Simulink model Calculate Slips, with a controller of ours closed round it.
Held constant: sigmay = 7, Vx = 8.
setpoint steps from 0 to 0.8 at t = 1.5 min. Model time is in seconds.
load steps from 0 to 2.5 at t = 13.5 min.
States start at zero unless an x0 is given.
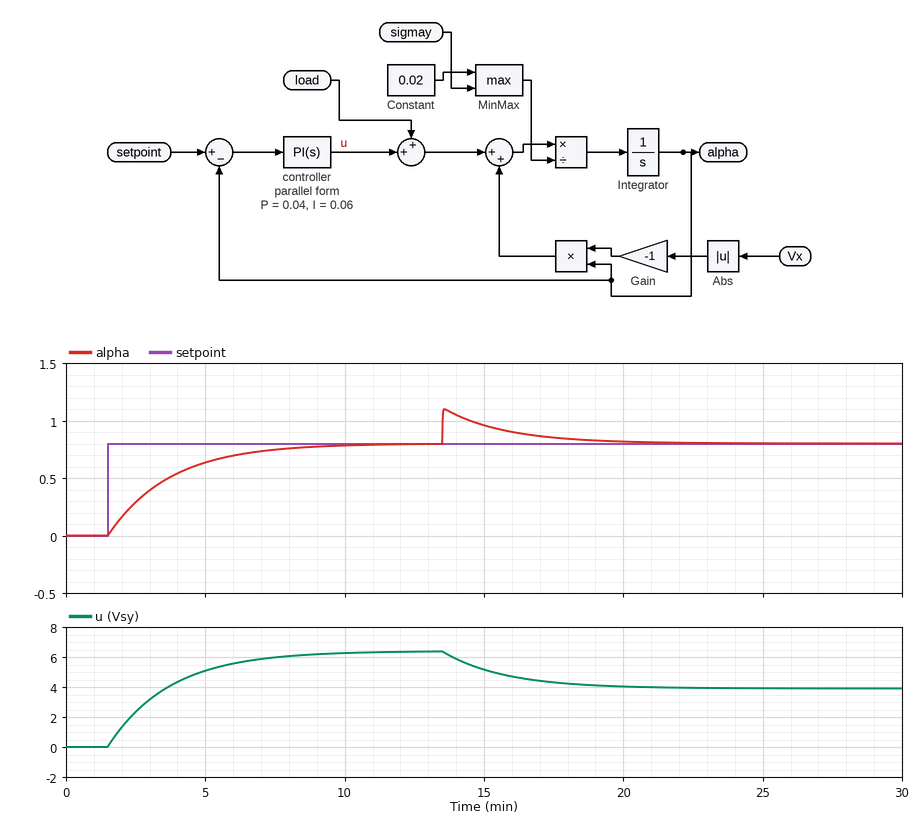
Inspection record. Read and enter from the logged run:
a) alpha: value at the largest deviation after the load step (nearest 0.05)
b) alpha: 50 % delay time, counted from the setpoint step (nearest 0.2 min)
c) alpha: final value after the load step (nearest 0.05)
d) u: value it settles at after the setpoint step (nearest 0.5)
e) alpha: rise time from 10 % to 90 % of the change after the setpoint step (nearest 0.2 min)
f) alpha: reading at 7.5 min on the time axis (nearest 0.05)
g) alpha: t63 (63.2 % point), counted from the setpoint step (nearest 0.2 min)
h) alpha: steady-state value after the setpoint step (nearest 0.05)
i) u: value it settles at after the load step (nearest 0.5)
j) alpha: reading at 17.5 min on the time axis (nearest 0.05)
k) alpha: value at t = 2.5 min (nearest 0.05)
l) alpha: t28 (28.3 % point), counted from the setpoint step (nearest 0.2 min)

1.10
1.6 min
0.80
6.5
4.8 min
0.75
2.2 min
0.80
4.0
0.85
0.30
0.8 min
